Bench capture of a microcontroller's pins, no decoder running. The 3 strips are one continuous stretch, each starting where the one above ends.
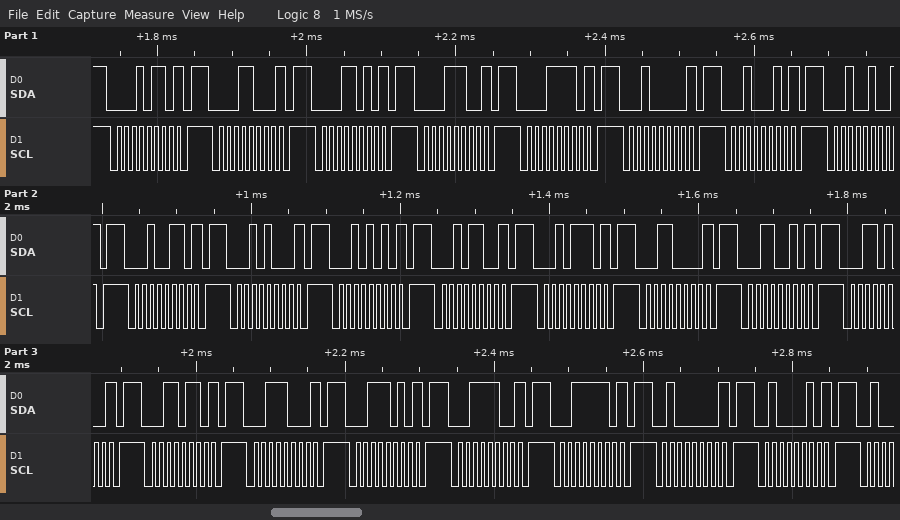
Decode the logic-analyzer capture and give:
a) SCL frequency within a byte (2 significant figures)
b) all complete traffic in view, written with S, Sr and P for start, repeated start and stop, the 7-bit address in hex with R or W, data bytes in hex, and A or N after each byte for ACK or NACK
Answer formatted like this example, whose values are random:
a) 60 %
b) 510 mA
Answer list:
a) 100 kHz
b) S 0BW N P S 0CW N P S 0DW N P S 0EW N P S 0FW N P S 10W N P S 11W N P S 12W N P S 13W N P S 14W N P S 15W N P S 16W N P S 17W N P S 18W N P S 19W N P S 1AW N P S 1BW N P S 1CW N P S 1DW N P S 1EW N P S 1FW N P S 20W N P S 21W N P
